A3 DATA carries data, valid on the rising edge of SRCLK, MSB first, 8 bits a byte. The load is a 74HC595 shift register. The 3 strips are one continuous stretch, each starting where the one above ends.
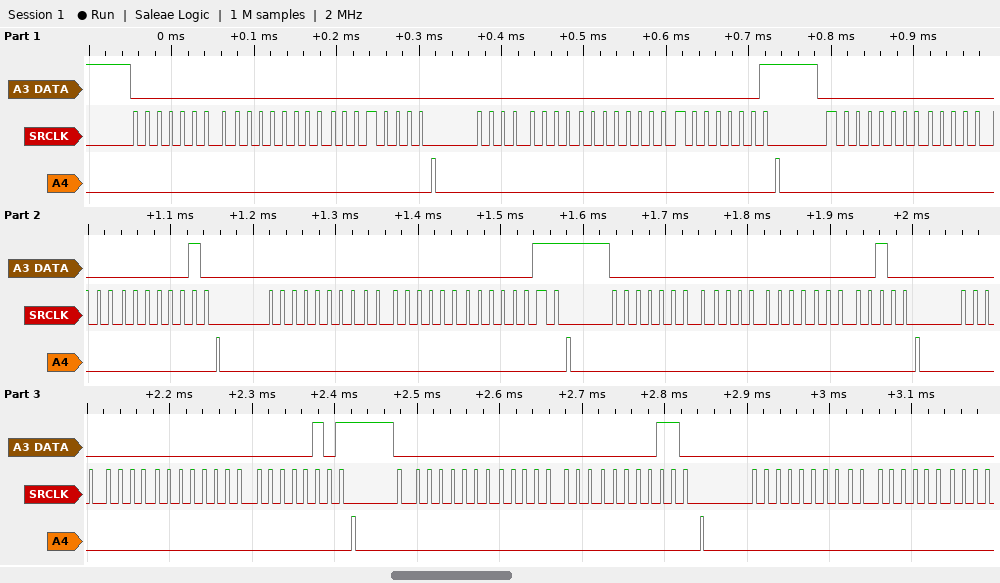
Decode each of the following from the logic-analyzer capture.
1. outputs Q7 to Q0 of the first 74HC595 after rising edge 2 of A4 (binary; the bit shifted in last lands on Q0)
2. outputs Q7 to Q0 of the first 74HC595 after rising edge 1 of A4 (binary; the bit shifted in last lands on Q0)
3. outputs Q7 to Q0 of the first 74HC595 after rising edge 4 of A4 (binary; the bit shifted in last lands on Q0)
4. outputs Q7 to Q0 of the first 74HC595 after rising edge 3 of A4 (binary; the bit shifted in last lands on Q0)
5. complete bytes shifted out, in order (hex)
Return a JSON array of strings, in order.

["00000001", "00000000", "00000011", "00000010", "00 00 00 00 00 01 00 00 02 00 00 03 00 00 04 00 00 05 00 00 06 00 00"]
